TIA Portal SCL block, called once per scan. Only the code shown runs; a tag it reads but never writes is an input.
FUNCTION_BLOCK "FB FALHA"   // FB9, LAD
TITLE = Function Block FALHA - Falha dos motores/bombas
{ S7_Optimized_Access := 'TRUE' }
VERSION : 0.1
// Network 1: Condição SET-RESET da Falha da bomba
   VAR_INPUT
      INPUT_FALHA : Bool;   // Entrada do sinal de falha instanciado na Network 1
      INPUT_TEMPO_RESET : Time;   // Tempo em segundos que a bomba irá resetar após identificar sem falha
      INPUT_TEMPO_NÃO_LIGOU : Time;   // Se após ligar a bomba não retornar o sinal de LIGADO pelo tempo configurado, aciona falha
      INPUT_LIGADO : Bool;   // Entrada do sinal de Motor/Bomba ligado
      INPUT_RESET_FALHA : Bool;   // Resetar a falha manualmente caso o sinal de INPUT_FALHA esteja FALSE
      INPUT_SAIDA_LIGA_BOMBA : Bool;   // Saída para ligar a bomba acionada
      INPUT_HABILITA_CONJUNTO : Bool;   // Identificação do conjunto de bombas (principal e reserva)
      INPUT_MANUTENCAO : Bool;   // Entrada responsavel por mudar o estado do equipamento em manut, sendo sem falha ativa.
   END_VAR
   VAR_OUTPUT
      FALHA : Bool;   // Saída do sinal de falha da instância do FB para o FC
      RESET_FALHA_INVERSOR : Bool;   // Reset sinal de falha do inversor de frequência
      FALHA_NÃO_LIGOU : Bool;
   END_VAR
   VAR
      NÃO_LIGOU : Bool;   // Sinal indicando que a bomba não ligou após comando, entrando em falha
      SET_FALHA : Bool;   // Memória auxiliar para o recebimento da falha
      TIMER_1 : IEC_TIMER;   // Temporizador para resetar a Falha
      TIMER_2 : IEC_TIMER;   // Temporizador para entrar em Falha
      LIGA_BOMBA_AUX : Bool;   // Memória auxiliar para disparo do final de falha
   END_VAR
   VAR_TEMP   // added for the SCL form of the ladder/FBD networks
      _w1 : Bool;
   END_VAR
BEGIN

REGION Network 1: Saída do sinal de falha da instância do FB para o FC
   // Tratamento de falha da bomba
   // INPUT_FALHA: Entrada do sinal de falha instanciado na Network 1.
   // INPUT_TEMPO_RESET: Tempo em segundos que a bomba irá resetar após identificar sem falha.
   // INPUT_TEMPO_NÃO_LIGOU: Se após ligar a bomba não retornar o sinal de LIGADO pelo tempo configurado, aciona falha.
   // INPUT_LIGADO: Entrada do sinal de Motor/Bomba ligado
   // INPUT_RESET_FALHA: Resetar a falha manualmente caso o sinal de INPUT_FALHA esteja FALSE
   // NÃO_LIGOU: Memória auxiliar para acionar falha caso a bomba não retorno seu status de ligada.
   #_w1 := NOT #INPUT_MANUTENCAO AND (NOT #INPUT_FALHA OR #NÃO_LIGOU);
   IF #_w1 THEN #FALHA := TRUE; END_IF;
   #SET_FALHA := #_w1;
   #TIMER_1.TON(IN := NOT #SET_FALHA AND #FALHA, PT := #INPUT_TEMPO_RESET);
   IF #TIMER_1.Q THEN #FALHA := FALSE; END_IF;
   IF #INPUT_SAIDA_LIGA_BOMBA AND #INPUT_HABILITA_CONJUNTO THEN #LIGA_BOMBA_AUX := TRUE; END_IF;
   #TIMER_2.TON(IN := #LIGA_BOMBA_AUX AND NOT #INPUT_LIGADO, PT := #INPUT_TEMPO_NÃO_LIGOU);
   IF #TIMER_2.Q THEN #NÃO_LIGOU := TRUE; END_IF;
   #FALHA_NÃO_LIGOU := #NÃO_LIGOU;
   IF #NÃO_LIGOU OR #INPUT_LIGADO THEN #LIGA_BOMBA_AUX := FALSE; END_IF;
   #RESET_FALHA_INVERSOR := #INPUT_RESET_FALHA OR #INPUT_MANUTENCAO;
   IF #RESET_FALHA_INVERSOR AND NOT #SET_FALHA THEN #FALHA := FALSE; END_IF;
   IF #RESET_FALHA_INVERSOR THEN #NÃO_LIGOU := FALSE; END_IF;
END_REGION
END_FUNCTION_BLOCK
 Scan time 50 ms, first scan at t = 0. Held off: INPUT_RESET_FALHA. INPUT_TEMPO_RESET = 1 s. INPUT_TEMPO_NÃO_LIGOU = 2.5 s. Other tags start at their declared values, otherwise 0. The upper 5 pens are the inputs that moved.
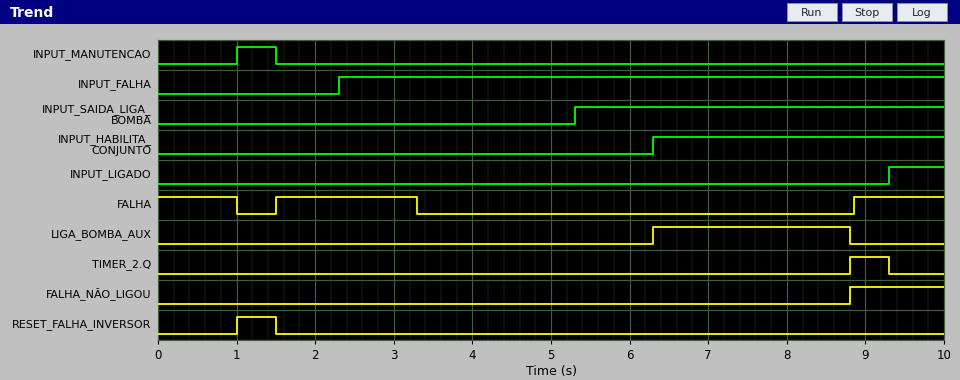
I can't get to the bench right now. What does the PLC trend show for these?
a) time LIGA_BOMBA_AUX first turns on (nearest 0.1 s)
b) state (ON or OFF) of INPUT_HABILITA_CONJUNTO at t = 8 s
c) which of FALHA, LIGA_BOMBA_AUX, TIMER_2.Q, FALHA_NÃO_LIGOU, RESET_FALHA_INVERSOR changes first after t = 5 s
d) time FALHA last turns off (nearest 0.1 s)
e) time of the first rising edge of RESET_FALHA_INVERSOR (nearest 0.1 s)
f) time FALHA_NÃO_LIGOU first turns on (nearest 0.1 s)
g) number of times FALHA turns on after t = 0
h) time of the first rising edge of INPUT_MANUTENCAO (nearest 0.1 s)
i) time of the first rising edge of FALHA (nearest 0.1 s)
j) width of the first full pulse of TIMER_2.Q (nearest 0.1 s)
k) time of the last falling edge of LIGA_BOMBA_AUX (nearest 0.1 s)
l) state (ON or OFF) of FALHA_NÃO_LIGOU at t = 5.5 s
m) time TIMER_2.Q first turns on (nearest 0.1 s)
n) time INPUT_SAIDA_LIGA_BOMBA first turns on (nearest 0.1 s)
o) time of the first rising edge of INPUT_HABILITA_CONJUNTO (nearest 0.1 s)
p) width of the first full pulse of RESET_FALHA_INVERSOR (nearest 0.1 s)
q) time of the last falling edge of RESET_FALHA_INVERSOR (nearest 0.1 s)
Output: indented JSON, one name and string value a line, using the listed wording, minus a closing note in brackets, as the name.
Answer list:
{
  "time LIGA_BOMBA_AUX first turns on": "6.3 s",
  "state (ON or OFF) of INPUT_HABILITA_CONJUNTO at t = 8 s": "ON",
  "which of FALHA, LIGA_BOMBA_AUX, TIMER_2.Q, FALHA_NÃO_LIGOU, RESET_FALHA_INVERSOR changes first after t = 5 s": "LIGA_BOMBA_AUX",
  "time FALHA last turns off": "3.3 s",
  "time of the first rising edge of RESET_FALHA_INVERSOR": "1.0 s",
  "time FALHA_NÃO_LIGOU first turns on": "8.8 s",
  "number of times FALHA turns on after t = 0": "2",
  "time of the first rising edge of INPUT_MANUTENCAO": "1.0 s",
  "time of the first rising edge of FALHA": "1.5 s",
  "width of the first full pulse of TIMER_2.Q": "0.5 s",
  "time of the last falling edge of LIGA_BOMBA_AUX": "8.8 s",
  "state (ON or OFF) of FALHA_NÃO_LIGOU at t = 5.5 s": "OFF",
  "time TIMER_2.Q first turns on": "8.8 s",
  "time INPUT_SAIDA_LIGA_BOMBA first turns on": "5.3 s",
  "time of the first rising edge of INPUT_HABILITA_CONJUNTO": "6.3 s",
  "width of the first full pulse of RESET_FALHA_INVERSOR": "0.5 s",
  "time of the last falling edge of RESET_FALHA_INVERSOR": "1.5 s"
}
